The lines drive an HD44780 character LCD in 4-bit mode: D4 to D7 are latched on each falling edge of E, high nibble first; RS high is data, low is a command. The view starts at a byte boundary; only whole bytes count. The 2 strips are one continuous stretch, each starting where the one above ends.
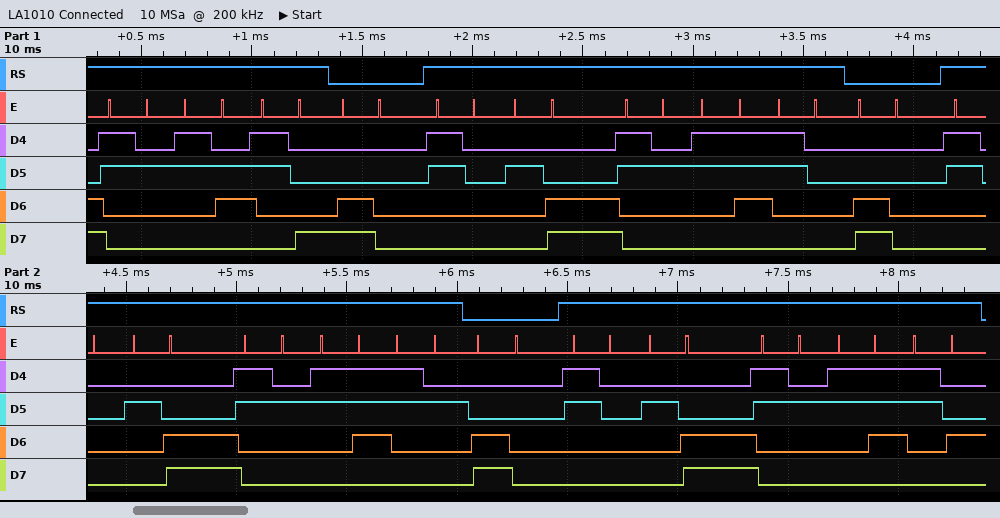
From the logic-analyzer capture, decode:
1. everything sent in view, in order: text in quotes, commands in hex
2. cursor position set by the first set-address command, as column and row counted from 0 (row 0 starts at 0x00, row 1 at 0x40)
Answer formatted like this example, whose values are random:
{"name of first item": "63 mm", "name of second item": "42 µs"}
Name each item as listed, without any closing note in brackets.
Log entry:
{"everything sent in view, in order: text in quotes, commands in hex": "\"268\" 0xC0 \"0,270\" 0xC0 \"0,272\" 0xC0 \"0,274\"", "cursor position set by the first set-address command, as column and row counted from 0": "column 0, row 1"}
